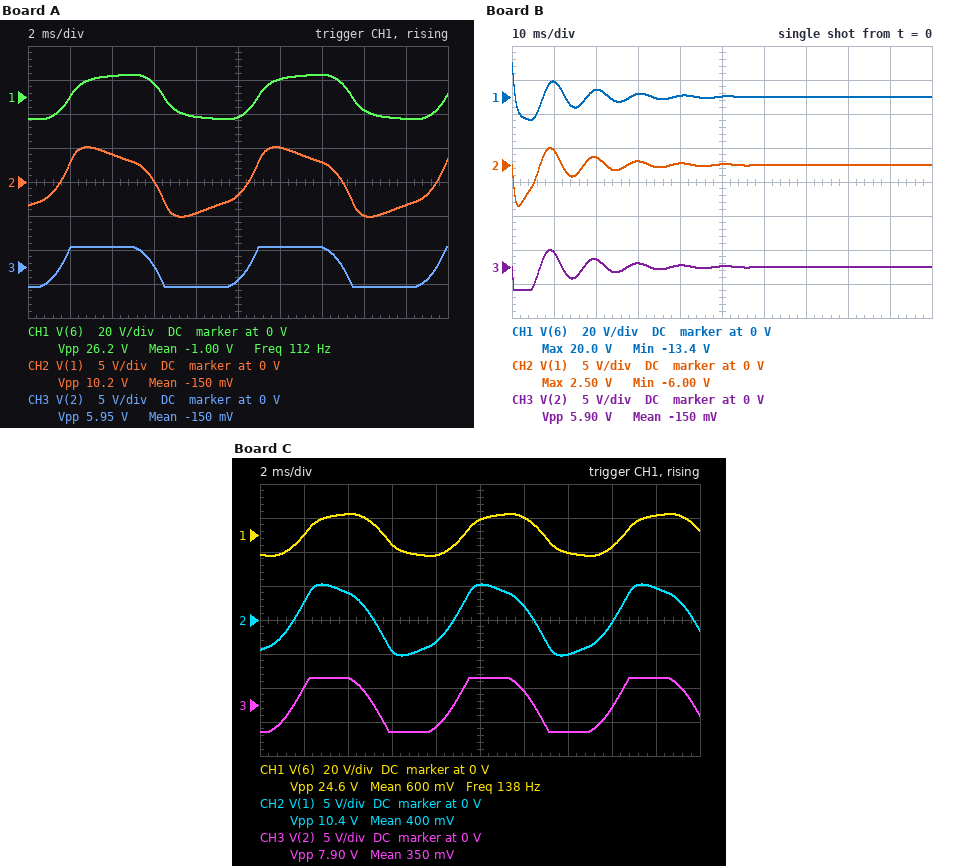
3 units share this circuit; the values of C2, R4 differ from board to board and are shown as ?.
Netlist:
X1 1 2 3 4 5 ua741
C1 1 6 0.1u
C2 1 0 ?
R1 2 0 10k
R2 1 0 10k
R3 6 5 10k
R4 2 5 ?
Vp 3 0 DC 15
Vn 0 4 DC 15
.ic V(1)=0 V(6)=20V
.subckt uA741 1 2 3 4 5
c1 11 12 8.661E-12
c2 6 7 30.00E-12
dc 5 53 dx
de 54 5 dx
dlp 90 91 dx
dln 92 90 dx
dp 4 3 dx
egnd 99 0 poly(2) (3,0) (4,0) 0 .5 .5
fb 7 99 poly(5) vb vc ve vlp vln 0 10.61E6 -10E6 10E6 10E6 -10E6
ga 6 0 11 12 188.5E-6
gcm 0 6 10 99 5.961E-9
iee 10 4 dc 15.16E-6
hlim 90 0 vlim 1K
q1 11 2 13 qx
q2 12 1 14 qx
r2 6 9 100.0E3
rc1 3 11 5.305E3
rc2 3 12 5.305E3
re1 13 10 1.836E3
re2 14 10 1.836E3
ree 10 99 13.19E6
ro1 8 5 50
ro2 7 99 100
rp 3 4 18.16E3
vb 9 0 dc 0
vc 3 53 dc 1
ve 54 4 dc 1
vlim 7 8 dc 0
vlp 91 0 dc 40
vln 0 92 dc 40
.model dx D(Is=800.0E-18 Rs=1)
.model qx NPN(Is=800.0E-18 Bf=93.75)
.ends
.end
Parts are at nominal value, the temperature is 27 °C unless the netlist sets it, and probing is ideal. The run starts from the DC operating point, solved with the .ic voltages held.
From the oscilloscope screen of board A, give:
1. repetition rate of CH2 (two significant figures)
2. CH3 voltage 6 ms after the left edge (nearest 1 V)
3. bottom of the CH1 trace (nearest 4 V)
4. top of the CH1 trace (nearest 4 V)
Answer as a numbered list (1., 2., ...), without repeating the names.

1. 110 Hz
2. 0 V
3. -12 V
4. 12 V
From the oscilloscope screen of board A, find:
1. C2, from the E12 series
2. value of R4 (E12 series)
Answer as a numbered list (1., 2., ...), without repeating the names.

1. 150 nF
2. 39 kΩ
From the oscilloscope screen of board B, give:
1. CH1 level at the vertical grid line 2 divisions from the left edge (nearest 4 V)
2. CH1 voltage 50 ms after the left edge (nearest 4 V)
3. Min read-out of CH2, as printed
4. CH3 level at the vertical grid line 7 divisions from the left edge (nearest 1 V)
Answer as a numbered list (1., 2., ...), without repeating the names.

1. 4 V
2. 0 V
3. -6.00 V
4. 0 V
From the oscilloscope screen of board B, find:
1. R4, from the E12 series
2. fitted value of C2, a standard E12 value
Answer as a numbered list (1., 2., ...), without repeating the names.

1. 33 kΩ
2. 270 nF
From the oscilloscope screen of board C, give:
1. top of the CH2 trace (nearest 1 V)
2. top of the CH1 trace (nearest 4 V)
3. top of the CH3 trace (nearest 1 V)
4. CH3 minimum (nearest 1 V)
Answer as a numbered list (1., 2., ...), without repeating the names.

1. 5 V
2. 12 V
3. 4 V
4. -4 V
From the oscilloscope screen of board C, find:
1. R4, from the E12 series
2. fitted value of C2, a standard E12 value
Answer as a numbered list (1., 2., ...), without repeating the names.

1. 27 kΩ
2. 120 nF
